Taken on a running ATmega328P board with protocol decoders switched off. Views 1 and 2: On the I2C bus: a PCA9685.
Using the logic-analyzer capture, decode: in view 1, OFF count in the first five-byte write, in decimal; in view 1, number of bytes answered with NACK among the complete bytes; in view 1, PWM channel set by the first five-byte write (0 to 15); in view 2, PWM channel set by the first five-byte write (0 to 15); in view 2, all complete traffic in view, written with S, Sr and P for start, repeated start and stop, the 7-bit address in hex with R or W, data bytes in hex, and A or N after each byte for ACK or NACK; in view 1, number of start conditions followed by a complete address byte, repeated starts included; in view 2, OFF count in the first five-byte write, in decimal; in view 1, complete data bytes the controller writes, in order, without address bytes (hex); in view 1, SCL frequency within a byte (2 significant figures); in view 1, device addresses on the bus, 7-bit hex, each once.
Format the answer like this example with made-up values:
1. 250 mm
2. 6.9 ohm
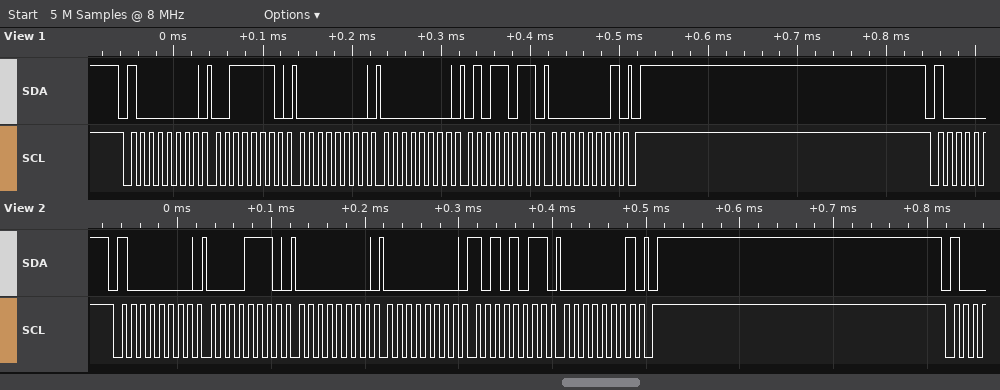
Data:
1. 347
2. 0
3. 14
4. 2
5. S 40W A 0E A 00 A 00 A AB A 01 A P
6. 1
7. 427
8. 3E 00 00 5B 01
9. 100 kHz
10. 0x40
